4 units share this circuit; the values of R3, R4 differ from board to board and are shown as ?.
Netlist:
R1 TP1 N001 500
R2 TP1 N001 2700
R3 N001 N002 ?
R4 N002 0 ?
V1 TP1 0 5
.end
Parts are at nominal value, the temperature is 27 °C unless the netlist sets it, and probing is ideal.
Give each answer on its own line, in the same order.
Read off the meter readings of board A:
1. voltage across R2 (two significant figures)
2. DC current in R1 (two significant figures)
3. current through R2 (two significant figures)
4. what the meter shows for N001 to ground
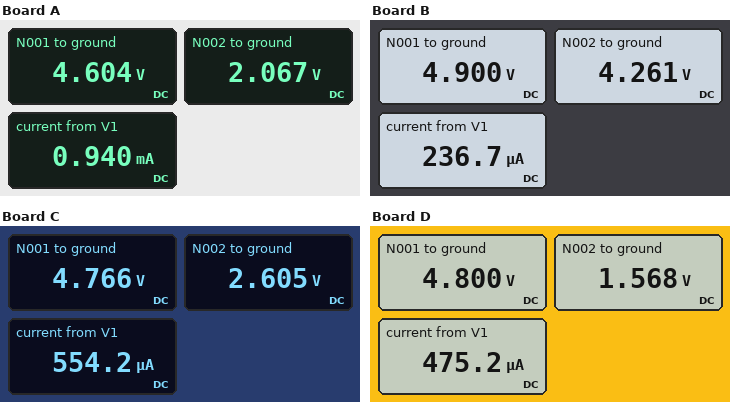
400 mV
790 µA
150 µA
4.604 V
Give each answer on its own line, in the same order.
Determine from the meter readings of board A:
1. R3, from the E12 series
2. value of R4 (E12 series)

2.7 kΩ
2.2 kΩ
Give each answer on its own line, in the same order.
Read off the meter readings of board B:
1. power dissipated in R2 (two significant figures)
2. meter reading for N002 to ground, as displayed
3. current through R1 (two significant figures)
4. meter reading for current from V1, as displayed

3.7 µW
4.261 V
200 µA
236.7 µA
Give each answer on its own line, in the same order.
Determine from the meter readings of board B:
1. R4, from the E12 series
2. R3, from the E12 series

18 kΩ
2.7 kΩ
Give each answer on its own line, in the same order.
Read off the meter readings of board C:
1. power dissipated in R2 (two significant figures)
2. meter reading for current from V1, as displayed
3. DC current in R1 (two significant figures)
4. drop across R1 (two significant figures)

20 µW
554.2 µA
470 µA
230 mV
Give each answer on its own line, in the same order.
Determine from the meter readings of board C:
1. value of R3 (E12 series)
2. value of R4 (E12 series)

3.9 kΩ
4.7 kΩ
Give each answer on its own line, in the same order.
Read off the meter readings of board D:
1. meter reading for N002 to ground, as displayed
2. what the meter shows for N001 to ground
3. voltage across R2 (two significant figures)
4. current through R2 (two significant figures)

1.568 V
4.800 V
200 mV
74 µA
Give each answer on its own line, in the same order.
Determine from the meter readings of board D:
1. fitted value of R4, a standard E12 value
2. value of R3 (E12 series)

3.3 kΩ
6.8 kΩ
